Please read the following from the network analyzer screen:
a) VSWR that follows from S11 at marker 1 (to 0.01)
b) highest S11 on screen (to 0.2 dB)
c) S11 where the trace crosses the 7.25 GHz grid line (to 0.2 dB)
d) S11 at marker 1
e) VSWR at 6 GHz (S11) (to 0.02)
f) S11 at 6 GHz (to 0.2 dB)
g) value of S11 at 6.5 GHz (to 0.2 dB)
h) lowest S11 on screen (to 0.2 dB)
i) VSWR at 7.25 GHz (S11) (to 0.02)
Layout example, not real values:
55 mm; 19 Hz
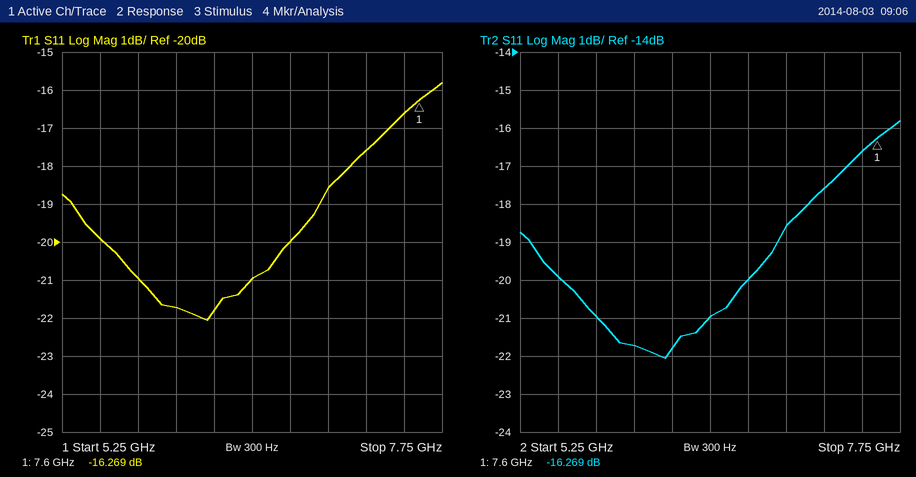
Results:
1.36; -15.8 dB; -17.6 dB; -16.269 dB; 1.18; -21.8 dB; -21.0 dB; -22.0 dB; 1.30
